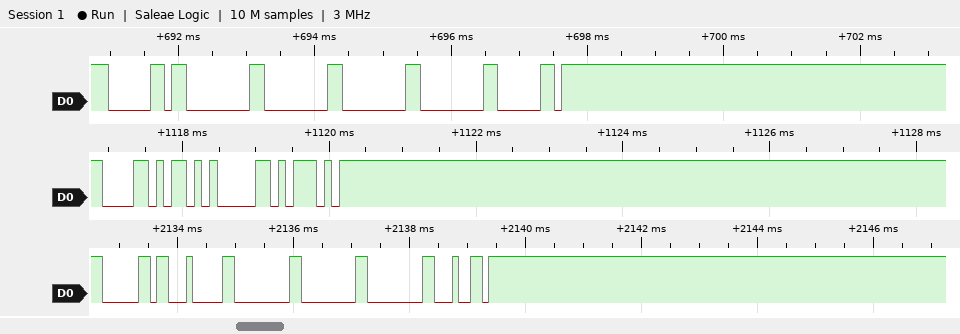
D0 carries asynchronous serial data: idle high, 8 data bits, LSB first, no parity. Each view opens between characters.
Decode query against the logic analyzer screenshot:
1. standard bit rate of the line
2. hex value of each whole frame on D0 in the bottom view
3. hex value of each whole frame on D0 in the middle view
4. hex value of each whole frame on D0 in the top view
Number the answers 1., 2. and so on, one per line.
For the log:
1. 9600 baud
2. 60, 04, 00, 00, 00, 64
3. 58, 05, 5D
4. 60, 00, 00, 00, 00, 60
